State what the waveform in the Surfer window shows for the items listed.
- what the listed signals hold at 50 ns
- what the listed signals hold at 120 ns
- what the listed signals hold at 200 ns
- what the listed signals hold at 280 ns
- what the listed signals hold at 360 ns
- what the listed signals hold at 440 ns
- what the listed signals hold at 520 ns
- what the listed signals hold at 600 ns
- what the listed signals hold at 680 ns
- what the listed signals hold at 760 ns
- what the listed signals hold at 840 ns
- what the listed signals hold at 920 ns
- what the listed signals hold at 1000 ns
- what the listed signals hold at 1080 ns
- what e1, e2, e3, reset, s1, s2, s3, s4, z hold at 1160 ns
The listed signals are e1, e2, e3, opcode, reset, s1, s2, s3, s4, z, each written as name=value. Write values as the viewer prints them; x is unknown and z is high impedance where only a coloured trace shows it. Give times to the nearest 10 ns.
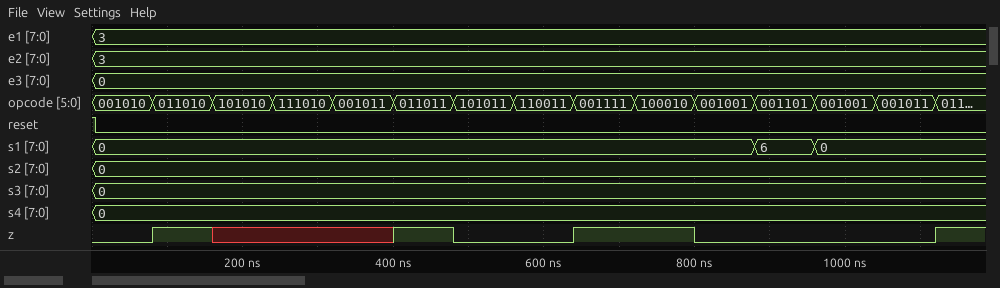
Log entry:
e1=3, e2=3, e3=0, opcode=001010, reset=0, s1=0, s2=0, s3=0, s4=0, z=0
e1=3, e2=3, e3=0, opcode=011010, reset=0, s1=0, s2=0, s3=0, s4=0, z=1
e1=3, e2=3, e3=0, opcode=101010, reset=0, s1=0, s2=0, s3=0, s4=0, z=x
e1=3, e2=3, e3=0, opcode=111010, reset=0, s1=0, s2=0, s3=0, s4=0, z=x
e1=3, e2=3, e3=0, opcode=001011, reset=0, s1=0, s2=0, s3=0, s4=0, z=x
e1=3, e2=3, e3=0, opcode=011011, reset=0, s1=0, s2=0, s3=0, s4=0, z=1
e1=3, e2=3, e3=0, opcode=101011, reset=0, s1=0, s2=0, s3=0, s4=0, z=0
e1=3, e2=3, e3=0, opcode=110011, reset=0, s1=0, s2=0, s3=0, s4=0, z=0
e1=3, e2=3, e3=0, opcode=001111, reset=0, s1=0, s2=0, s3=0, s4=0, z=1
e1=3, e2=3, e3=0, opcode=100010, reset=0, s1=0, s2=0, s3=0, s4=0, z=1
e1=3, e2=3, e3=0, opcode=001001, reset=0, s1=0, s2=0, s3=0, s4=0, z=0
e1=3, e2=3, e3=0, opcode=001101, reset=0, s1=6, s2=0, s3=0, s4=0, z=0
e1=3, e2=3, e3=0, opcode=001001, reset=0, s1=0, s2=0, s3=0, s4=0, z=0
e1=3, e2=3, e3=0, opcode=001011, reset=0, s1=0, s2=0, s3=0, s4=0, z=0
e1=3, e2=3, e3=0, reset=0, s1=0, s2=0, s3=0, s4=0, z=1
